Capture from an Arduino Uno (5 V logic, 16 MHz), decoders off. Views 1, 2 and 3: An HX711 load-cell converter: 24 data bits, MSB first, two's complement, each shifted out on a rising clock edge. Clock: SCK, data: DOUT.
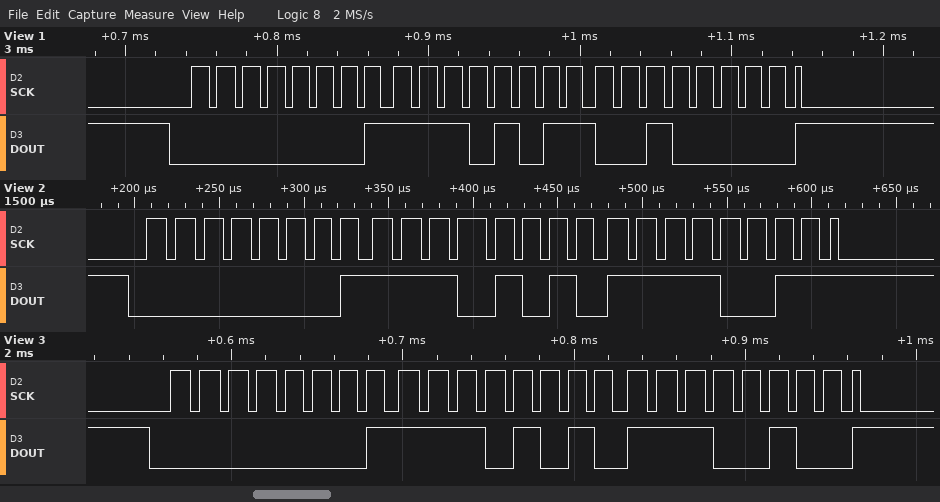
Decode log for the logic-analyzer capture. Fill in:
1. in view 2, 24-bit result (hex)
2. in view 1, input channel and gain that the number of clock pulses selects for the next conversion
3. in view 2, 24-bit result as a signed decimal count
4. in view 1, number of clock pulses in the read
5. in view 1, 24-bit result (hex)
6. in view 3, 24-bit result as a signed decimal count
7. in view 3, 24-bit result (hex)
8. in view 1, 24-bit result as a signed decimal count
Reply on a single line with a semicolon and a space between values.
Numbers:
0x01EAF3; channel A, gain 128; 125683; 25; 0x01EB20; 125668; 0x01EAE4; 125728
